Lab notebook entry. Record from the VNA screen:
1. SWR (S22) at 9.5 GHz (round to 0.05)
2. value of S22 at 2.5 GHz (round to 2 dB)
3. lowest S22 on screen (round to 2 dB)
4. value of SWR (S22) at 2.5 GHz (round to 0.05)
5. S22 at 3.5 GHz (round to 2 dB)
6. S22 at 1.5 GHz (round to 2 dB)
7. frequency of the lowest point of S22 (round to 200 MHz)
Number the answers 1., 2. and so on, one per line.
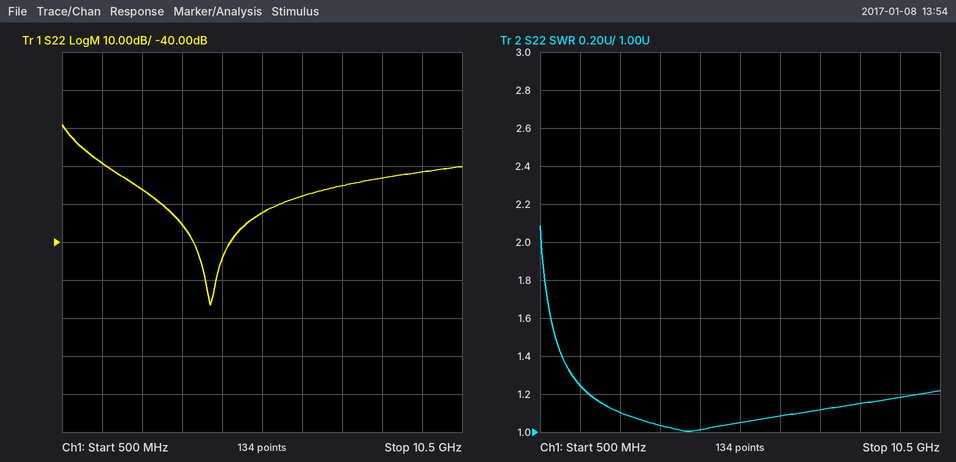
1. 1.20
2. -26 dB
3. -56 dB
4. 1.10
5. -36 dB
6. -20 dB
7. 4.2 GHz
